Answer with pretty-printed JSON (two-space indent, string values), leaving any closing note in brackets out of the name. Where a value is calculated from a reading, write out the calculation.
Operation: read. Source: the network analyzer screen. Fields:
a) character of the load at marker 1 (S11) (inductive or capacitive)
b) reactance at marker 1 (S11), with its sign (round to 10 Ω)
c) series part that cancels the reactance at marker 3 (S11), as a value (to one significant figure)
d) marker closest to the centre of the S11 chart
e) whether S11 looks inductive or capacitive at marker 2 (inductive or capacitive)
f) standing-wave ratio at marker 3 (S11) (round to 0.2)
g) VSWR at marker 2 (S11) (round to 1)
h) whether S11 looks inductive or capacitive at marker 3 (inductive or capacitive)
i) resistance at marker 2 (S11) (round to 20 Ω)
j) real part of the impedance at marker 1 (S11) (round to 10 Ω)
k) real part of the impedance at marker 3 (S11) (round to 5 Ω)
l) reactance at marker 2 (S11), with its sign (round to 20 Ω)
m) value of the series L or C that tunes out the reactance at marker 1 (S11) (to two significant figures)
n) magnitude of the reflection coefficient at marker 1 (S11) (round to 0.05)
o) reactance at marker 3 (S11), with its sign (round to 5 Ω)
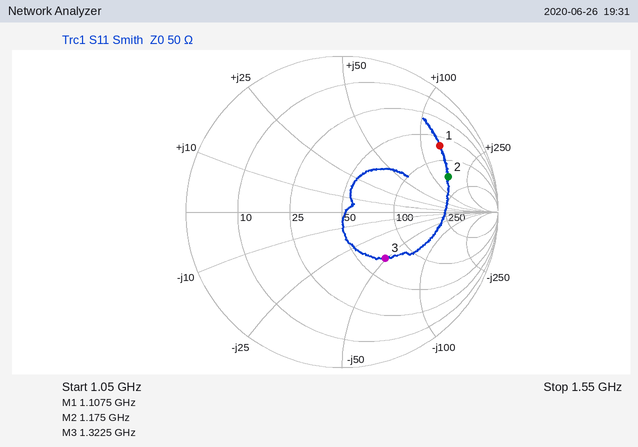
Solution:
{
  "character of the load at marker 1 (S11)": "inductive",
  "reactance at marker 1 (S11), with its sign": "+130 Ω",
  "series part that cancels the reactance at marker 3 (S11), as a value": "L = 50 Ω/(2π × 1.3225 GHz) ≈ 6 nH",
  "marker closest to the centre of the S11 chart": "marker 3",
  "whether S11 looks inductive or capacitive at marker 2": "inductive",
  "standing-wave ratio at marker 3 (S11)": "2.4",
  "VSWR at marker 2 (S11)": "6",
  "whether S11 looks inductive or capacitive at marker 3": "capacitive",
  "resistance at marker 2 (S11)": "160 Ω",
  "real part of the impedance at marker 1 (S11)": "70 Ω",
  "real part of the impedance at marker 3 (S11)": "70 Ω",
  "reactance at marker 2 (S11), with its sign": "+140 Ω",
  "value of the series L or C that tunes out the reactance at marker 1 (S11)": "C = 1/(2π × 1.1075 GHz × 130 Ω) ≈ 1.1 pF",
  "magnitude of the reflection coefficient at marker 1 (S11)": "0.75",
  "reactance at marker 3 (S11), with its sign": "-50 Ω"
}
